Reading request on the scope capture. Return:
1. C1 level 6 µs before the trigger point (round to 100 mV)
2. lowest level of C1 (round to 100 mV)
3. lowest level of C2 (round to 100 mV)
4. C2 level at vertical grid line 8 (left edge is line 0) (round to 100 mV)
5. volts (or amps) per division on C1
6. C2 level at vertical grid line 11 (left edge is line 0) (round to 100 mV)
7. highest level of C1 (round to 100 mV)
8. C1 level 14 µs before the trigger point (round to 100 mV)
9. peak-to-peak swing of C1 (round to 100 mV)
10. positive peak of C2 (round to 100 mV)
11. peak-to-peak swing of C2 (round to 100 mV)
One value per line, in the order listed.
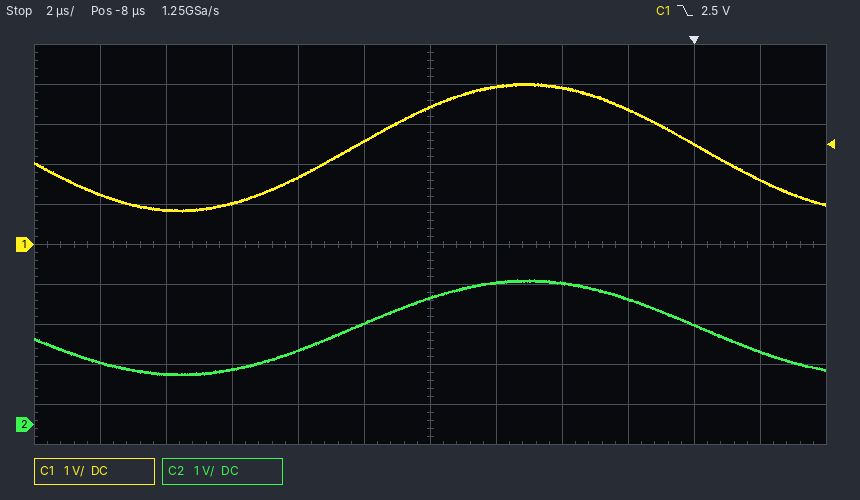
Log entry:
3.9 V
800 mV
1.2 V
3.5 V
1 V
1.8 V
4.0 V
1.0 V
3.2 V
3.6 V
2.4 V
